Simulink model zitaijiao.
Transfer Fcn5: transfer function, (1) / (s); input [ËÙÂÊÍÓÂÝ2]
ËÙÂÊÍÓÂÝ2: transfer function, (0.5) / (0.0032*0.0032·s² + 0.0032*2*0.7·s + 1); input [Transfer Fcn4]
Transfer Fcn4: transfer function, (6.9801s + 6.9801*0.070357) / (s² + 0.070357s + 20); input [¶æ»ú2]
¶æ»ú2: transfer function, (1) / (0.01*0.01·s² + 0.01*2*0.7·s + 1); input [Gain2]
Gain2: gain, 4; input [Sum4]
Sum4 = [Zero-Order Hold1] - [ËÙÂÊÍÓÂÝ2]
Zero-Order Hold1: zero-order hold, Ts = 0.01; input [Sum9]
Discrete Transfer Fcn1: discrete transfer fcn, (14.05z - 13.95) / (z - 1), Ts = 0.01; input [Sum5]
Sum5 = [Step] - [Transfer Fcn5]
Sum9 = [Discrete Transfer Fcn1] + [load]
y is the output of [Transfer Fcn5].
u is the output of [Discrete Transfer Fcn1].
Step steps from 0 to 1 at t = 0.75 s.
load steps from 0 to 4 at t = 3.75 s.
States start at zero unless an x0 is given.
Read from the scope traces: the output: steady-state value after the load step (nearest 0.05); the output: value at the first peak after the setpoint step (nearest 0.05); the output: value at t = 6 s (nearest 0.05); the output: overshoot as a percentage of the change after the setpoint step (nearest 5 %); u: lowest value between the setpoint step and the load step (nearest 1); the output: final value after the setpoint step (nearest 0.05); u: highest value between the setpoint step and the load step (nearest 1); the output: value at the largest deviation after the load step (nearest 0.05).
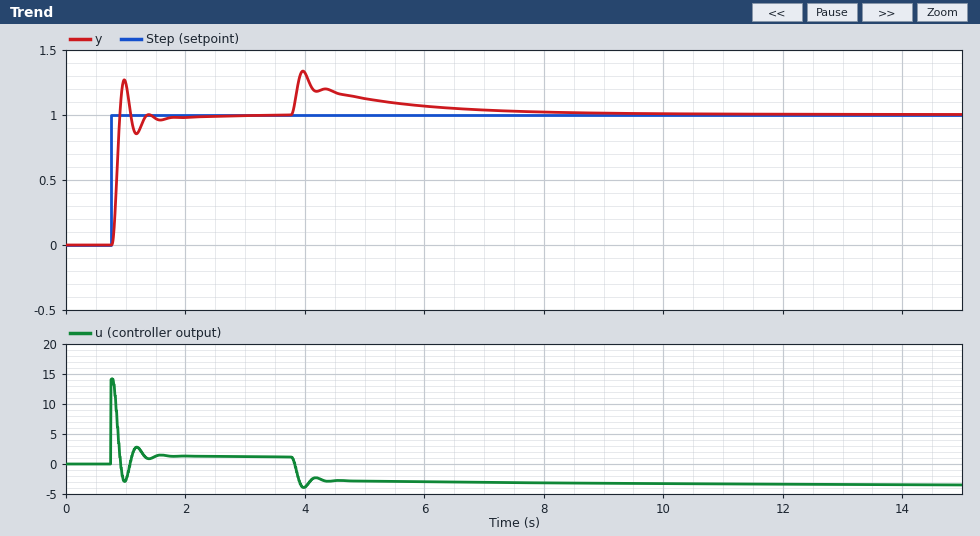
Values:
1.00
1.25
1.05
25 %
-3
1.00
14
1.35
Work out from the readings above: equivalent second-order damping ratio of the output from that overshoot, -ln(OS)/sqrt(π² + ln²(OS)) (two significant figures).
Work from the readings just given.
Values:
0.40
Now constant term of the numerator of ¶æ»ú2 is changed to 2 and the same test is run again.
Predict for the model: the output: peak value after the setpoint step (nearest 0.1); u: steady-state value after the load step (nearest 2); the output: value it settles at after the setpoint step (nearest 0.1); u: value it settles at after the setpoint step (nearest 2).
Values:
1.1
-4
1.0
0
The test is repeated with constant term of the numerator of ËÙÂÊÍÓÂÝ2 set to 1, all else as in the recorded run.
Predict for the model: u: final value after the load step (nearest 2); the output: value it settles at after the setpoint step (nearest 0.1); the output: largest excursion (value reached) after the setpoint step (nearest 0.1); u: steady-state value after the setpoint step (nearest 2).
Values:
-4
1.0
1.1
0
